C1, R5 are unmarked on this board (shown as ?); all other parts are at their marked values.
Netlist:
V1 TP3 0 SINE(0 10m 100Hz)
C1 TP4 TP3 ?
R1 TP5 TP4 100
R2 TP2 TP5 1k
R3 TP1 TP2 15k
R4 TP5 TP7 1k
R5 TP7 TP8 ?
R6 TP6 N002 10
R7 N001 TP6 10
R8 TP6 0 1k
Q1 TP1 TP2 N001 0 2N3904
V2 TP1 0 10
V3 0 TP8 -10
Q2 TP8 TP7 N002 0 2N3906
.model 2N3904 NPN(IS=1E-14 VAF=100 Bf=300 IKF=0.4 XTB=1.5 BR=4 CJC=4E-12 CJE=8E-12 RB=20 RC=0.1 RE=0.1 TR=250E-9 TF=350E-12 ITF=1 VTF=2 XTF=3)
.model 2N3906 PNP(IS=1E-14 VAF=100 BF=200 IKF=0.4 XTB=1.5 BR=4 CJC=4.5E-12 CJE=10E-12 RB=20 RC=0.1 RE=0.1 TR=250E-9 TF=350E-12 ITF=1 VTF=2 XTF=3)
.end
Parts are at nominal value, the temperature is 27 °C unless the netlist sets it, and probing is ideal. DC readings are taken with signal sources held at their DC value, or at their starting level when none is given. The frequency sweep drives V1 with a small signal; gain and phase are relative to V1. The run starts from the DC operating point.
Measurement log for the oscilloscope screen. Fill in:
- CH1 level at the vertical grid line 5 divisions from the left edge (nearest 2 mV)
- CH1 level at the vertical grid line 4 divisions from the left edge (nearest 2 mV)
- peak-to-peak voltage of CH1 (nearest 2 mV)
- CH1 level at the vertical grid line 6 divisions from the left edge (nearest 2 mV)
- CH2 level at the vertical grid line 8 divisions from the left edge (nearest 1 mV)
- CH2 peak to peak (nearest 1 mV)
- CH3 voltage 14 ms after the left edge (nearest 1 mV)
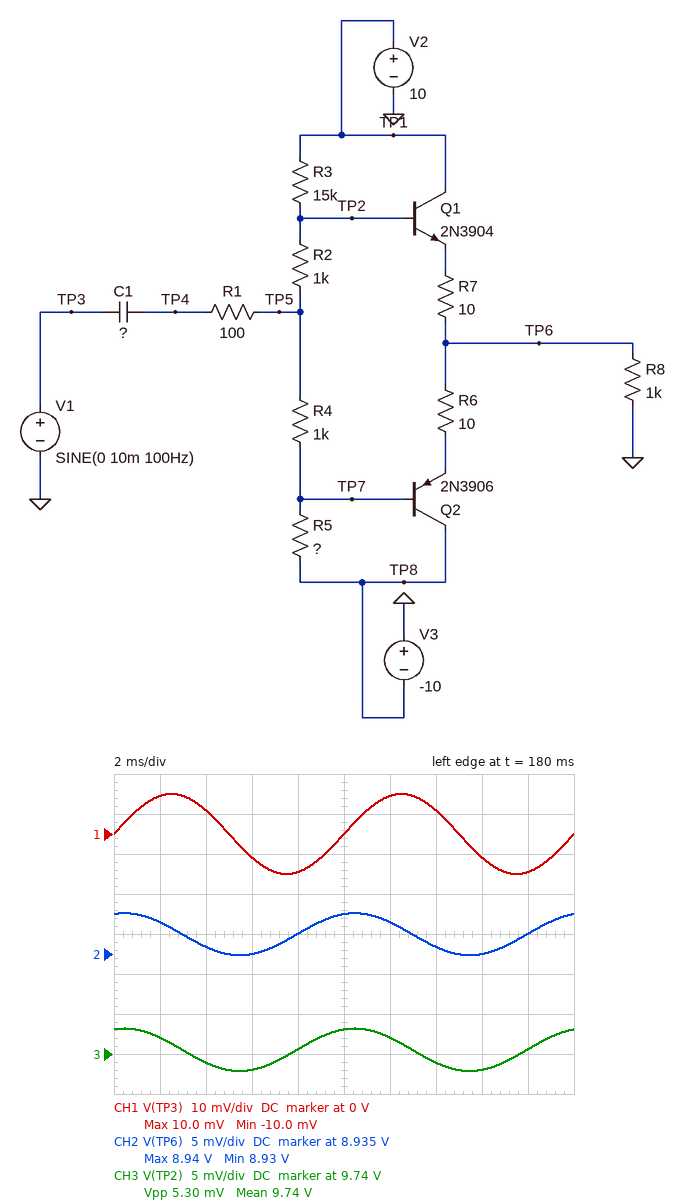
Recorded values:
0 V
-10 mV
20 mV
10 mV
8.935 V
5 mV
9.739 V
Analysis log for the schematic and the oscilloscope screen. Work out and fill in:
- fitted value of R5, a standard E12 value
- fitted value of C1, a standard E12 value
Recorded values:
18 kΩ
56 nF
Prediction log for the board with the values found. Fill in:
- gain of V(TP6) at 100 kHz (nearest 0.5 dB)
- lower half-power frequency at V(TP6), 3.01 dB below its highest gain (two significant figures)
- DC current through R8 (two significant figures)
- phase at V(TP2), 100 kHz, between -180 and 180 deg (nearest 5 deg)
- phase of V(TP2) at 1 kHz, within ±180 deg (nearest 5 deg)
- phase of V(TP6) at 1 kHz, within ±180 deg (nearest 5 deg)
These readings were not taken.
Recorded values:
-1.0 dB
330 Hz
8.9 mA
0 deg
20 deg
20 deg
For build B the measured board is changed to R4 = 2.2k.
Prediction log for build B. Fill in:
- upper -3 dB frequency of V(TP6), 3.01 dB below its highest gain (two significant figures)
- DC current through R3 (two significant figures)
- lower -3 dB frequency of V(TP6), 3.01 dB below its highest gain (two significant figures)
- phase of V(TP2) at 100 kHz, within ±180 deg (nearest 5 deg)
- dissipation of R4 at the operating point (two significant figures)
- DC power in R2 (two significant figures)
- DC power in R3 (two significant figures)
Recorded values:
38 MHz
18 µA
320 Hz
0 deg
350 nW
160 nW
4.7 µW
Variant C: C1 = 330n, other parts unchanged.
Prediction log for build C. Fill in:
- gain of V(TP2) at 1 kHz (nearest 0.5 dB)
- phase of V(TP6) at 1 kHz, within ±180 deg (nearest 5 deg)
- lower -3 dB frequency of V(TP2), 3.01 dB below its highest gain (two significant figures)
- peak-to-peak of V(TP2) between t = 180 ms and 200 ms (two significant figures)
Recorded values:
-0.5 dB
5 deg
56 Hz
16 mV
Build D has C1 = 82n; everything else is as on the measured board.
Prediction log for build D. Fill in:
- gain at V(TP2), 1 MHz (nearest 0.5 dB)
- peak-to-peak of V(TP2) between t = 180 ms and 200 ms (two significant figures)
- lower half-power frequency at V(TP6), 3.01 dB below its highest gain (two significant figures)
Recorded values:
-0.5 dB
7.4 mV
230 Hz
